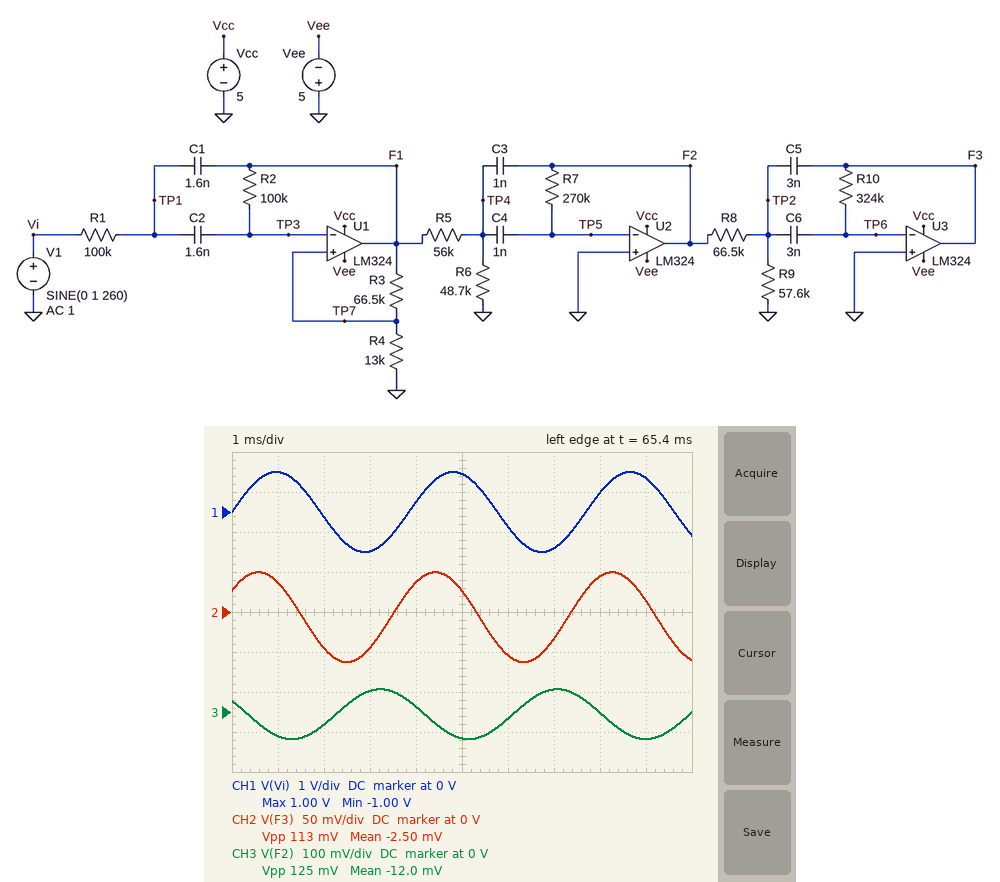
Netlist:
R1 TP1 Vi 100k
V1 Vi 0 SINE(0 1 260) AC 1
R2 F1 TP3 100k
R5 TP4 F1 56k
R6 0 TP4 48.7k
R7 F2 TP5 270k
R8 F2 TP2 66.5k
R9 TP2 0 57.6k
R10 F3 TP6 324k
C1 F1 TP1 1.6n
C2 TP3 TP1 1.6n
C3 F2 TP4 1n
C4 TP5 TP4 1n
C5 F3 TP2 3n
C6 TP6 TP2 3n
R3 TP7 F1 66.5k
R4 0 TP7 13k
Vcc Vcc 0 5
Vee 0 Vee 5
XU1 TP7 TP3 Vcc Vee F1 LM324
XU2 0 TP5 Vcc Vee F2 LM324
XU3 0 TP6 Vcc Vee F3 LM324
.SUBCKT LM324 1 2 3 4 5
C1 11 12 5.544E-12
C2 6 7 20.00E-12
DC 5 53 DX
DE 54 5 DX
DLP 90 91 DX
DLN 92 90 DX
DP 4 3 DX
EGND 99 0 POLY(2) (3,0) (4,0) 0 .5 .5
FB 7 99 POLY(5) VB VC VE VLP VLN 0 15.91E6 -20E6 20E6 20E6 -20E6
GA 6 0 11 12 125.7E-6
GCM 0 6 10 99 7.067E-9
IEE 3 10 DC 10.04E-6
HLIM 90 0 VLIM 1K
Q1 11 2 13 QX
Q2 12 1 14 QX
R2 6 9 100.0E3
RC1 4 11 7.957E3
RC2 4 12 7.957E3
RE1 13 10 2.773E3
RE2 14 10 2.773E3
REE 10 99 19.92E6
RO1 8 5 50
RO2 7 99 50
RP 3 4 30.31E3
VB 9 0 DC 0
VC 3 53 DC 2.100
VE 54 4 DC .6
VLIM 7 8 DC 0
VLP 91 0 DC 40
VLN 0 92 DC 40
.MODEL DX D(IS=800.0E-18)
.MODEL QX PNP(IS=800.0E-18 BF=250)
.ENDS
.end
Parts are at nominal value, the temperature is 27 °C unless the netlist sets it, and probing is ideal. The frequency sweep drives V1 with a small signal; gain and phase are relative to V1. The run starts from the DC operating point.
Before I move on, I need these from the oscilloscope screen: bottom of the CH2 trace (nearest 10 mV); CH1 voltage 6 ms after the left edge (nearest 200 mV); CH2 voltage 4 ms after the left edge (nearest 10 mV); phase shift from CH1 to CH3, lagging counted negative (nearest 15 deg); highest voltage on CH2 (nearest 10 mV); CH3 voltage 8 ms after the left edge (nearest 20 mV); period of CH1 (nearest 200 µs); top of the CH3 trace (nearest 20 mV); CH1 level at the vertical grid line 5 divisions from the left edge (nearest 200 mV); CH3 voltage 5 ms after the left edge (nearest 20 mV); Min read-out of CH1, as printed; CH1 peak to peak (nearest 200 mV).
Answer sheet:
-60 mV
-400 mV
40 mV
150 deg
50 mV
0 V
3.8 ms
60 mV
1.0 V
-60 mV
-1.00 V
2.0 V
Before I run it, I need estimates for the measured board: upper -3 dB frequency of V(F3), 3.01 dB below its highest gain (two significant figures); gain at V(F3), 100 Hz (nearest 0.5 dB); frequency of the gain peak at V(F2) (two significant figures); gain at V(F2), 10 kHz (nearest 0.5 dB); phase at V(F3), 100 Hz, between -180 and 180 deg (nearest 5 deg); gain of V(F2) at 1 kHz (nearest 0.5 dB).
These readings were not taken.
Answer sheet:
2.0 kHz
-51.0 dB
1.8 kHz
-29.5 dB
70 deg
-3.5 dB
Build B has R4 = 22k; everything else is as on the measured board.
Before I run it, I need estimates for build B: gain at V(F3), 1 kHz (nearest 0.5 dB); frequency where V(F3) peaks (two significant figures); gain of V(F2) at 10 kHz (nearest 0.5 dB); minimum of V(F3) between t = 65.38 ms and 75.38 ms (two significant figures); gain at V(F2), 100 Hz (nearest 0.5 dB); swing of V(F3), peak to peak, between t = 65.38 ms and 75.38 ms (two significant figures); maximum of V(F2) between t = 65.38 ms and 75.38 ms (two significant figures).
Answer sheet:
-2.0 dB
710 Hz
-28.5 dB
-70 mV
-39.5 dB
130 mV
65 mV
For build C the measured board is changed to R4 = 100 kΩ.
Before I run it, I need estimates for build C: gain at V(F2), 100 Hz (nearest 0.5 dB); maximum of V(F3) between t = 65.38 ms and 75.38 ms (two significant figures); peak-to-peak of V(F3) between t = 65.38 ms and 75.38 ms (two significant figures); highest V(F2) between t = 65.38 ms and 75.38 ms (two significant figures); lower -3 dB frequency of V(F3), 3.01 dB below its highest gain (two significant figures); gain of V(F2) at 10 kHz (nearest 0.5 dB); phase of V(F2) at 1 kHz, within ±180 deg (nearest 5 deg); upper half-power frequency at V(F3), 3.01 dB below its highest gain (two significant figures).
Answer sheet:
-34.0 dB
120 mV
260 mV
140 mV
750 Hz
-23.0 dB
65 deg
1.3 kHz
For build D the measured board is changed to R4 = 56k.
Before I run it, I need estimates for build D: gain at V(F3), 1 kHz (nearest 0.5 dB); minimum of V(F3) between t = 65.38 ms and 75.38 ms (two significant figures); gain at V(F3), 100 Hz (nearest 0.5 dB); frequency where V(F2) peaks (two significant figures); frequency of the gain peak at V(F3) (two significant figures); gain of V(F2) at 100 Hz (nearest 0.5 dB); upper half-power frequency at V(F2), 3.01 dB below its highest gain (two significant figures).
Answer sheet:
4.0 dB
-99 mV
-47.5 dB
1.7 kHz
980 Hz
-36.5 dB
2.2 kHz
